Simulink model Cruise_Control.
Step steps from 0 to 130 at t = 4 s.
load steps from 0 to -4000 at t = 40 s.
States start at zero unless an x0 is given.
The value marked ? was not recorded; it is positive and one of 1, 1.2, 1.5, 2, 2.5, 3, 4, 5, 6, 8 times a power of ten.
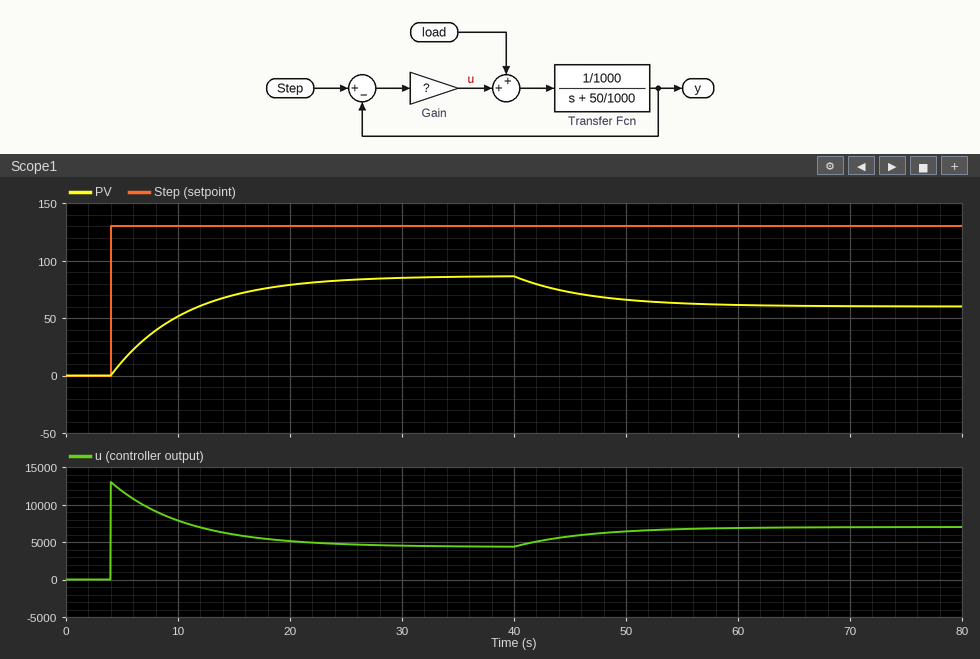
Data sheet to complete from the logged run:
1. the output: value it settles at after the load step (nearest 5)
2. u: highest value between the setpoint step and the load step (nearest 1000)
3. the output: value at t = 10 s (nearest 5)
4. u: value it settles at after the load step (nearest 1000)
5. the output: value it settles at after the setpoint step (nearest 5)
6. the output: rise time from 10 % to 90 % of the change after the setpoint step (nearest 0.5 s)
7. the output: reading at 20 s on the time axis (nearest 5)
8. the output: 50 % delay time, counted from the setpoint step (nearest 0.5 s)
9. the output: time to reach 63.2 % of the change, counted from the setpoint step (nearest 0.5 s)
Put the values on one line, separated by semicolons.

60; 13000; 50; 7000; 85; 14.5 s; 80; 4.5 s; 6.5 s
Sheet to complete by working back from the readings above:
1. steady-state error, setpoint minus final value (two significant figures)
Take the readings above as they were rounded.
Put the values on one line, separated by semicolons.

45
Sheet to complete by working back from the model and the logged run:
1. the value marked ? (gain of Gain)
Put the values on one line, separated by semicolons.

100
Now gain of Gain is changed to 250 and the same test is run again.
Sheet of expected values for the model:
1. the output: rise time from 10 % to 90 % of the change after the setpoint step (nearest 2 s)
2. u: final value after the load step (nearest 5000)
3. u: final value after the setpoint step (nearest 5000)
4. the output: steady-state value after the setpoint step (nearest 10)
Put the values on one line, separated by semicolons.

8 s; 10000; 5000; 110
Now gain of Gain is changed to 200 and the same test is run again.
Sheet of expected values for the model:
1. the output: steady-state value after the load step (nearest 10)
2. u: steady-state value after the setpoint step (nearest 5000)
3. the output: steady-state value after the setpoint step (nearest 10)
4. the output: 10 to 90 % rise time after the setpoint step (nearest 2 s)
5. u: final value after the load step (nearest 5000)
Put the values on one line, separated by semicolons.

90; 5000; 100; 8 s; 10000
